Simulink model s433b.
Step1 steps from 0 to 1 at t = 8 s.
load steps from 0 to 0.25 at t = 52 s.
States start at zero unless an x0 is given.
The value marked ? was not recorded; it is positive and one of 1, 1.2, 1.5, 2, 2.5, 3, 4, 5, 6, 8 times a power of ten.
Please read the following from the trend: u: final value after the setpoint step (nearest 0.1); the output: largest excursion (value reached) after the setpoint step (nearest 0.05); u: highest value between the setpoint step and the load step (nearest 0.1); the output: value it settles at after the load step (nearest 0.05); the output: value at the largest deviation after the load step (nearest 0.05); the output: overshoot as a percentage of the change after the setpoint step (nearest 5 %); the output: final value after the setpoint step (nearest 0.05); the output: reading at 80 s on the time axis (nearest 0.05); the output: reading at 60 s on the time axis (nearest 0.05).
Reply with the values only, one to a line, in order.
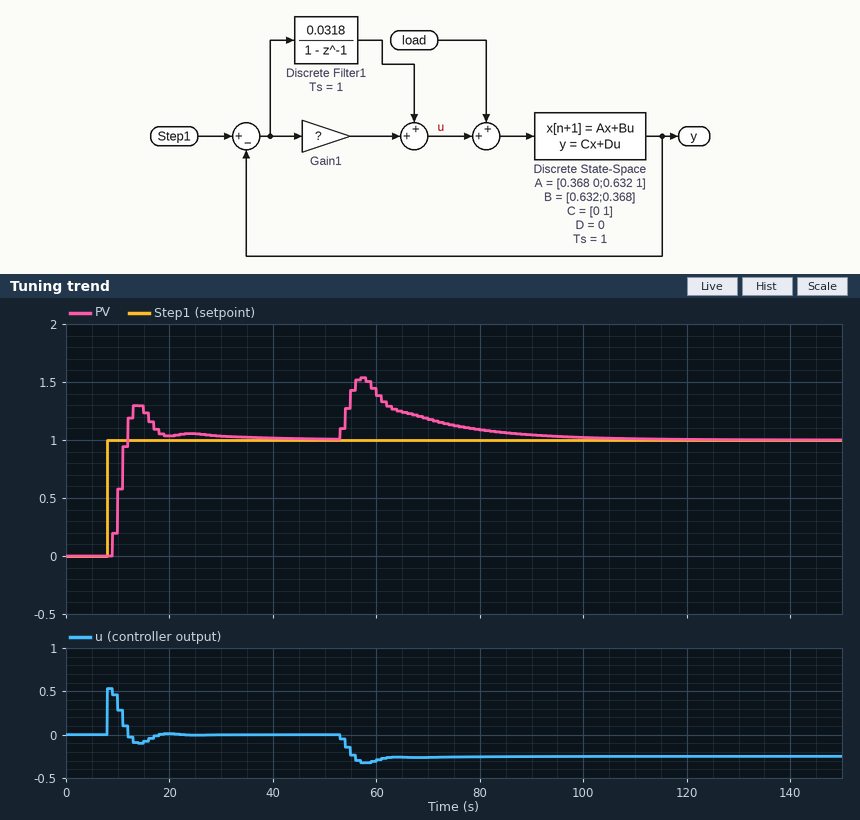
0.0
1.30
0.5
1.00
1.55
30 %
1.00
1.10
1.40
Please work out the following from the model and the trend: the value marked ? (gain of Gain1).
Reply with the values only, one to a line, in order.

0.5
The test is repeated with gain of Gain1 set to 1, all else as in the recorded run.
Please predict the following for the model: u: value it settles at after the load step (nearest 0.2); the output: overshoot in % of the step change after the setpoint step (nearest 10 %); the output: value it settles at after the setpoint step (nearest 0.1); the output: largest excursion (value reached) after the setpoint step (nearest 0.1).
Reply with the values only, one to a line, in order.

-0.2
50 %
1.0
1.5
